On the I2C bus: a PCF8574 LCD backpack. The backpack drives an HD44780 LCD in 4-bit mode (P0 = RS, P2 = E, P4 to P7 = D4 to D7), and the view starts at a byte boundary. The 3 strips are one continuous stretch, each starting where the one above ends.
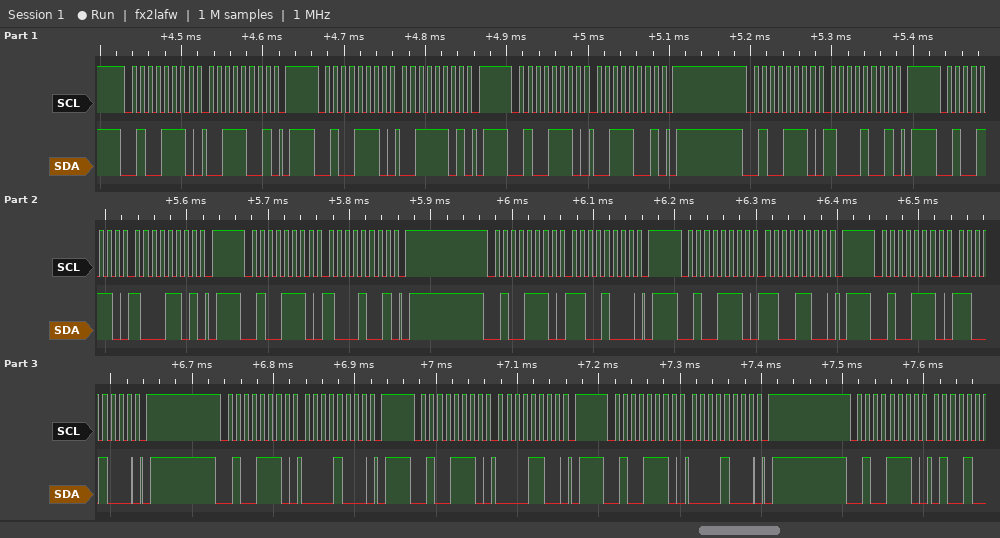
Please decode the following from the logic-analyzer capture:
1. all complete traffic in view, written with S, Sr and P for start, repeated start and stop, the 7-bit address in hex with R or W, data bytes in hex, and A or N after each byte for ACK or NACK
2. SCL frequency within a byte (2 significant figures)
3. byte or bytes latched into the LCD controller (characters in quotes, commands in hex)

S 27W A 39 A P S 27W A 3D A P S 27W A 39 A P S 27W A 89 A P S 27W A 8D A P S 27W A 89 A P S 27W A C8 A P S 27W A CC A P S 27W A C8 A P S 27W A 08 A P S 27W A 0C A P S 27W A 08 A P S 27W A
100 kHz
'8' 0xC0
